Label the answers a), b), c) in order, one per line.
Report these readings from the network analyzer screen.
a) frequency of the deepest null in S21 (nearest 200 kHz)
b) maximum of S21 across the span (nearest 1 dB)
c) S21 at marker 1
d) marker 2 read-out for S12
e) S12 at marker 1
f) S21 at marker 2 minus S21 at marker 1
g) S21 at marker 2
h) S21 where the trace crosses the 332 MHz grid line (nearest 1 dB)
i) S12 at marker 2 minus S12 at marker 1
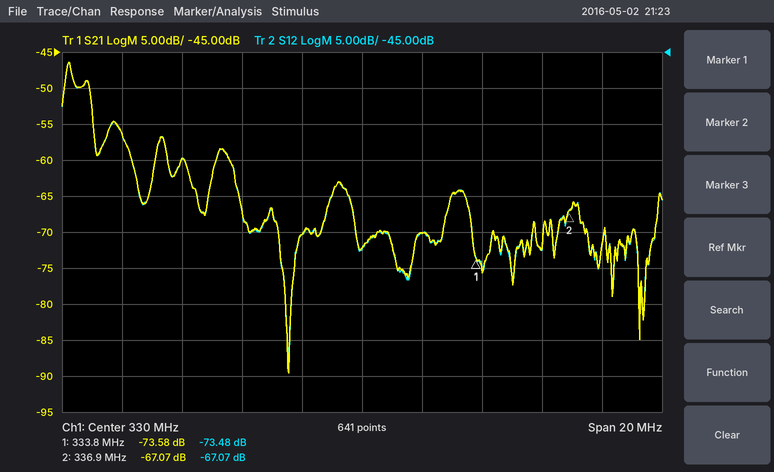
a) 327.6 MHz
b) -46 dB
c) -73.58 dB
d) -67.07 dB
e) -73.48 dB
f) 6.51 dB
g) -67.07 dB
h) -70 dB
i) 6.41 dB
